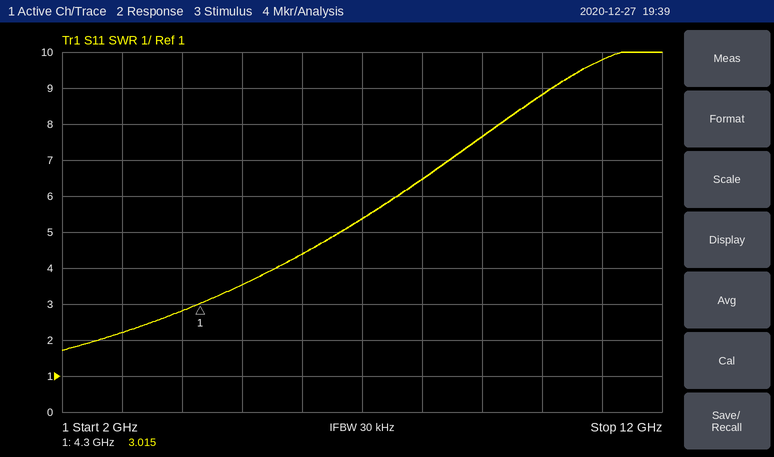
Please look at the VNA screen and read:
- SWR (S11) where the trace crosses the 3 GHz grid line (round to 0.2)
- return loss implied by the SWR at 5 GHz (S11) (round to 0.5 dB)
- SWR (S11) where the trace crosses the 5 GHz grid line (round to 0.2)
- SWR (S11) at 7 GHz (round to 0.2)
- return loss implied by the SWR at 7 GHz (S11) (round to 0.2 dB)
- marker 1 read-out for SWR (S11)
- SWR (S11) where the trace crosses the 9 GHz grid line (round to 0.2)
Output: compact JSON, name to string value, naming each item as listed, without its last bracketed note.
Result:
{"SWR (S11) where the trace crosses the 3 GHz grid line": "2.2", "return loss implied by the SWR at 5 GHz (S11)": "5.0 dB", "SWR (S11) where the trace crosses the 5 GHz grid line": "3.6", "SWR (S11) at 7 GHz": "5.4", "return loss implied by the SWR at 7 GHz (S11)": "3.2 dB", "marker 1 read-out for SWR": "3.015", "SWR (S11) where the trace crosses the 9 GHz grid line": "7.6"}
